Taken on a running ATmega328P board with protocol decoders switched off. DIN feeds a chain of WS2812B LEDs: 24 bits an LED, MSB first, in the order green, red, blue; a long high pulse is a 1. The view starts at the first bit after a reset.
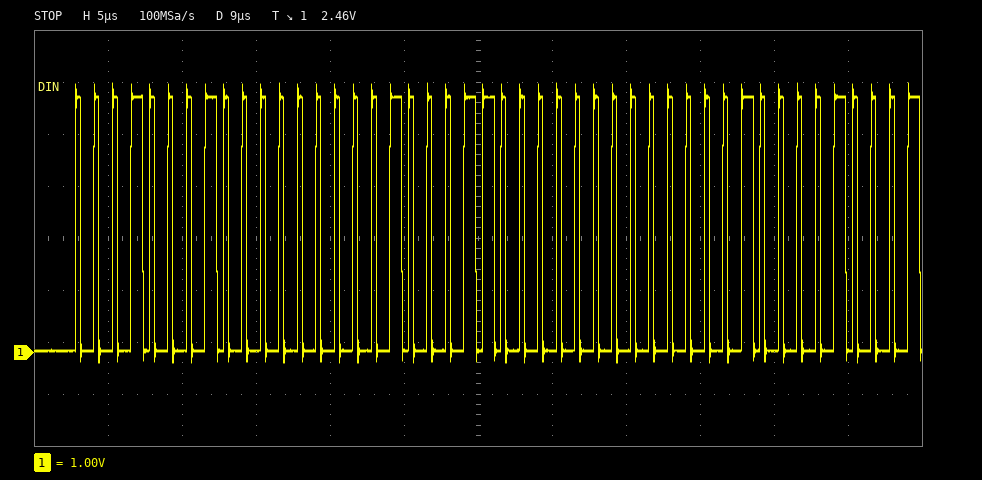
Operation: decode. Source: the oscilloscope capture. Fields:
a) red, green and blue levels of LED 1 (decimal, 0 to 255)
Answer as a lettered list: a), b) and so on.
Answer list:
a) 0, 17, 70
